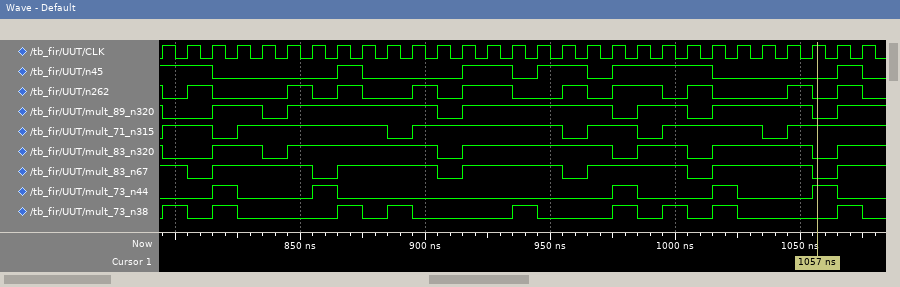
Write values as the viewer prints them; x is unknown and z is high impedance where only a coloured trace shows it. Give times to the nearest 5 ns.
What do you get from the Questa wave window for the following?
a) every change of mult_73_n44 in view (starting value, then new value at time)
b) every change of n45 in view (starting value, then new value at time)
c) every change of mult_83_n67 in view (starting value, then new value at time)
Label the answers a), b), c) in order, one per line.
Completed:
a) 0, 1 at 815 ns, 0 at 825 ns, 1 at 855 ns, 0 at 865 ns, 1 at 975 ns, 0 at 985 ns, 1 at 1015 ns, 0 at 1025 ns, 1 at 1055 ns, 0 at 1065 ns
b) 1, 0 at 815 ns, 1 at 865 ns, 0 at 875 ns, 1 at 915 ns, 0 at 935 ns, 1 at 945 ns, 0 at 965 ns, 1 at 975 ns, 0 at 1015 ns, 1 at 1065 ns, 0 at 1075 ns
c) 1, 0 at 805 ns, 1 at 815 ns, 0 at 855 ns, 1 at 865 ns, 0 at 905 ns, 1 at 915 ns, 0 at 955 ns, 1 at 965 ns, 0 at 1005 ns, 1 at 1015 ns, 0 at 1055 ns, 1 at 1065 ns
